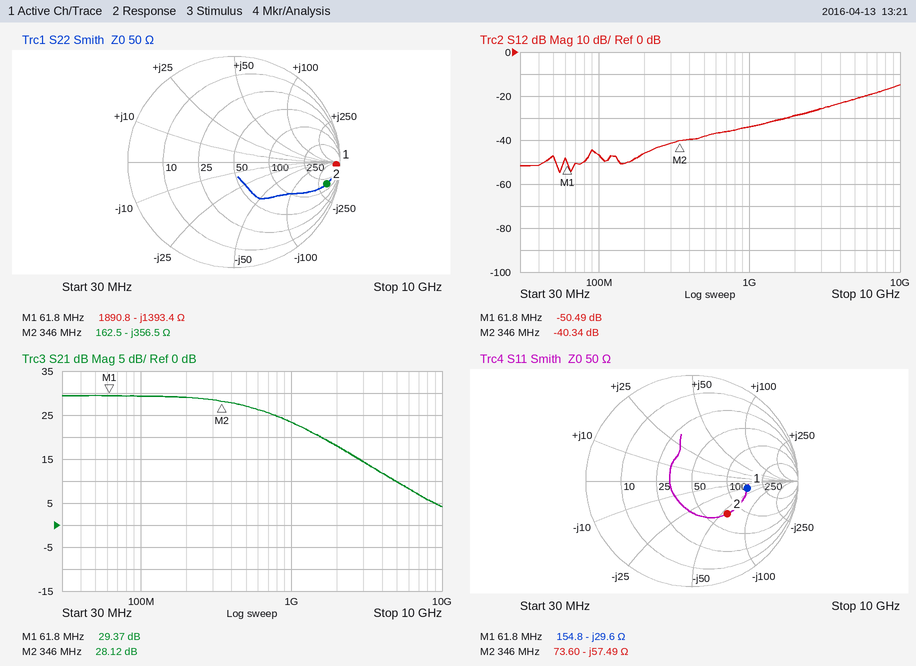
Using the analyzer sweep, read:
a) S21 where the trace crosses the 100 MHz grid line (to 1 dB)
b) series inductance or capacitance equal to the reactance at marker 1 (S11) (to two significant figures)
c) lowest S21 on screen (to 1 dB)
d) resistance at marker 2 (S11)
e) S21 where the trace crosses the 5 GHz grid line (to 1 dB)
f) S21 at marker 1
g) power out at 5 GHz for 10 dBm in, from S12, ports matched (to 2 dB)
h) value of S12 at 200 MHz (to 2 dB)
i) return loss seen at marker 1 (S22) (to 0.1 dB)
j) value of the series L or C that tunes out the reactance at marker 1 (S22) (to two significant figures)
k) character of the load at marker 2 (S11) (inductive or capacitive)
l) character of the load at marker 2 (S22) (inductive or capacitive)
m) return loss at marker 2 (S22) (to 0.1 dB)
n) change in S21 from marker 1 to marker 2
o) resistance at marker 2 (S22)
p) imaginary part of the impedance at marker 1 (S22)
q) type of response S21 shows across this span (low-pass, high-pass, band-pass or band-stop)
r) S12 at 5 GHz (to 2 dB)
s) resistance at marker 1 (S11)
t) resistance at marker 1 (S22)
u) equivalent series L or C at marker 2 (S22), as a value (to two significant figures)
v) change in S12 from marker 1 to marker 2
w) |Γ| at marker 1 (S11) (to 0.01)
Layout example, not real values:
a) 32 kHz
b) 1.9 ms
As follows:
a) 29 dB
b) 87 pF
c) 4 dB
d) 73.60 Ω
e) 10 dB
f) 29.37 dB
g) -12 dBm
h) -46 dB
i) 0.3 dB
j) 3.6 µH
k) capacitive
l) capacitive
m) 0.9 dB
n) -1.25 dB
o) 162.5 Ω
p) -1393.4 Ω
q) low-pass
r) -22 dB
s) 154.8 Ω
t) 1890.8 Ω
u) 1.3 pF
v) 10.15 dB
w) 0.53
